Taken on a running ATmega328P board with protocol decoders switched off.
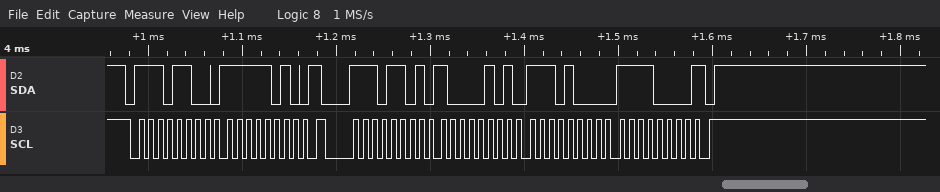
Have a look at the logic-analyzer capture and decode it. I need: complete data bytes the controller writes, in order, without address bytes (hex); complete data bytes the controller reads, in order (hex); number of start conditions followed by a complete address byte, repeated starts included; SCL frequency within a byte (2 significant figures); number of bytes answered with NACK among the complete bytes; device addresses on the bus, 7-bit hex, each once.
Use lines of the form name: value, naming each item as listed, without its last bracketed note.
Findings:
complete data bytes the controller writes, in order, without address bytes: FA
complete data bytes the controller reads, in order: 85 E8 F0
number of start conditions followed by a complete address byte, repeated starts included: 2
SCL frequency within a byte: 100 kHz
number of bytes answered with NACK among the complete bytes: 1
device addresses on the bus, 7-bit hex, each once: 0x76
